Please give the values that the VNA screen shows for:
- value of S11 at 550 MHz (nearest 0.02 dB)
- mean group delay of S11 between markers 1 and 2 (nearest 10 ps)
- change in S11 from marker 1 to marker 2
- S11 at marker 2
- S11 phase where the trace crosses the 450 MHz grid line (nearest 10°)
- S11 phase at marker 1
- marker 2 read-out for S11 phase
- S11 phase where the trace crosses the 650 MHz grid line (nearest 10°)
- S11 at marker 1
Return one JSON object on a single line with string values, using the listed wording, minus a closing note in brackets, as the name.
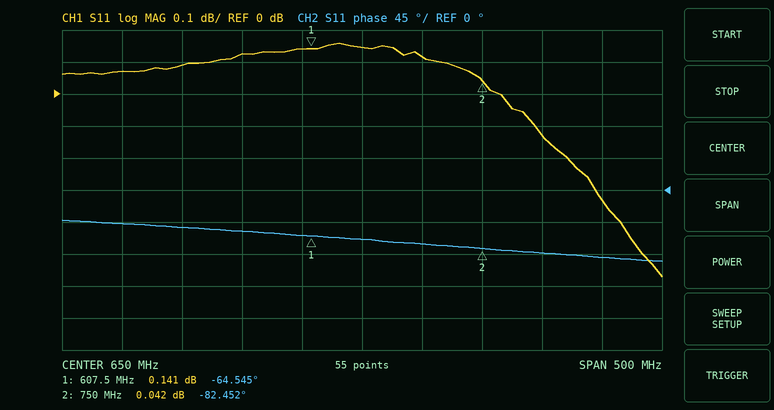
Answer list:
{"value of S11 at 550 MHz": "0.12 dB", "mean group delay of S11 between markers 1 and 2": "350 ps", "change in S11 from marker 1 to marker 2": "-0.099 dB", "S11 at marker 2": "0.042 dB", "S11 phase where the trace crosses the 450 MHz grid line": "-50°", "S11 phase at marker 1": "-64.545°", "marker 2 read-out for S11 phase": "-82.452°", "S11 phase where the trace crosses the 650 MHz grid line": "-70°", "S11 at marker 1": "0.141 dB"}
